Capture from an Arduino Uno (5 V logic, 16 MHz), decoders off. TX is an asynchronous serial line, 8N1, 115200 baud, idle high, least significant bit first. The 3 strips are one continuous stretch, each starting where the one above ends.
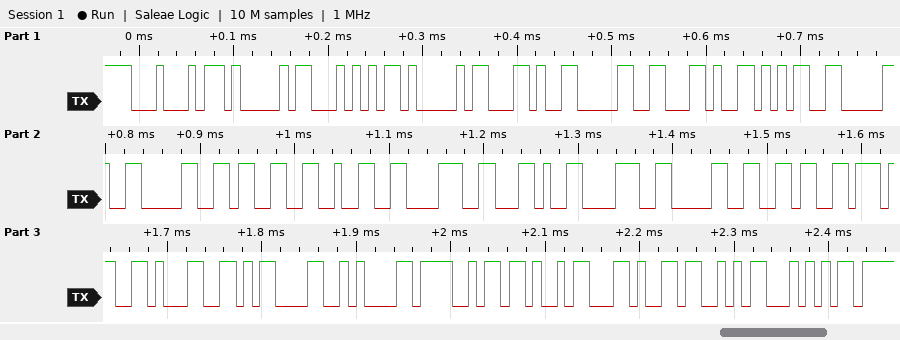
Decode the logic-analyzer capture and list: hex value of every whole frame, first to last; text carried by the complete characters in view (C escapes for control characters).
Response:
44 41 54 41 2C 30 2C 35 30 30 33 32 38 2C 38 30 36 37 31 0D 0A 4F 4B 2C 53 54
"DATA,0,500328,80671\r\nOK,ST"
